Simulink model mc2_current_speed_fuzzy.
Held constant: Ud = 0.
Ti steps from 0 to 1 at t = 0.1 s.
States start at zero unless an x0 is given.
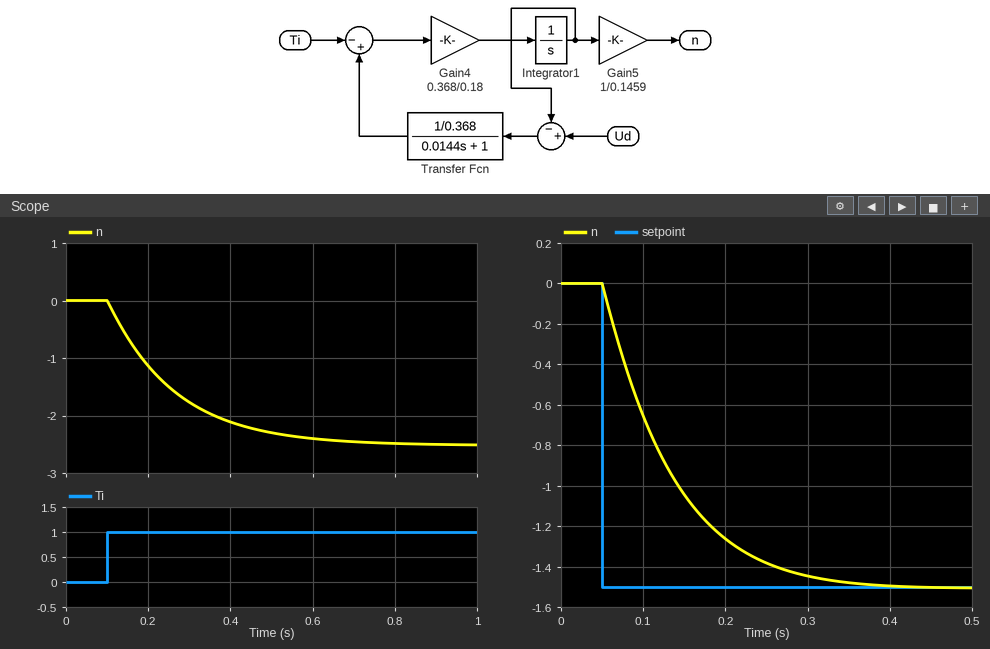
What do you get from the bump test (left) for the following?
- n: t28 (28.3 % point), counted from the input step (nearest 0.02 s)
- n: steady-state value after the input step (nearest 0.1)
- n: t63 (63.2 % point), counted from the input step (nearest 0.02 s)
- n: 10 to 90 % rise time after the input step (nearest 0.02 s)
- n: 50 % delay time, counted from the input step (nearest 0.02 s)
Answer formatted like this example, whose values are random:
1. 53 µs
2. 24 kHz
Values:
1. 0.06 s
2. -2.5
3. 0.16 s
4. 0.36 s
5. 0.12 s
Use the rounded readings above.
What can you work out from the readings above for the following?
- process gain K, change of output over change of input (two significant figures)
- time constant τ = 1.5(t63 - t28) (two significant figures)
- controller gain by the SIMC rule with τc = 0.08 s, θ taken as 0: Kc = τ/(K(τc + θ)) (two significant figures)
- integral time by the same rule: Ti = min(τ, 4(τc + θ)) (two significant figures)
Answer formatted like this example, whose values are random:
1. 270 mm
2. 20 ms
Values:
1. -2.5
2. 0.15 s
3. -0.75
4. 0.15 s
